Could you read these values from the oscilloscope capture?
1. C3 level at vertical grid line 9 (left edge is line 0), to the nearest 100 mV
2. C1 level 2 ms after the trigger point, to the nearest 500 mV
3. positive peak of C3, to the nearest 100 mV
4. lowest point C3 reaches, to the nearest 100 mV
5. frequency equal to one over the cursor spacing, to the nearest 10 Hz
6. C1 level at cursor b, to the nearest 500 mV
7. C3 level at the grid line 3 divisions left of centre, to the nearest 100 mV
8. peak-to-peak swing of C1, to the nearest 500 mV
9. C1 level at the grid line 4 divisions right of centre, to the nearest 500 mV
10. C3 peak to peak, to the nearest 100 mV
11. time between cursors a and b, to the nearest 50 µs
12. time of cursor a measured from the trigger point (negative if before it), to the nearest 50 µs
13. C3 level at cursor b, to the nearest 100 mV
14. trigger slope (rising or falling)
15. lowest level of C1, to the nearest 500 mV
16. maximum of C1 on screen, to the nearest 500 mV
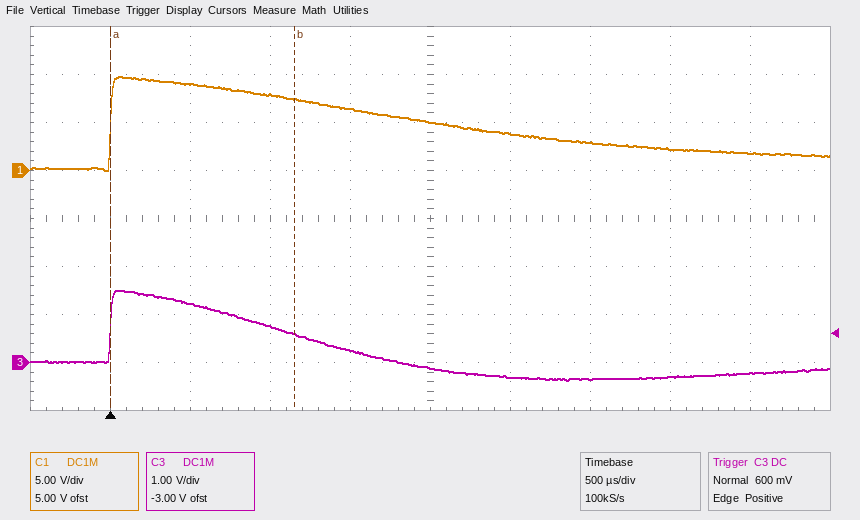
-200 mV
5.0 V
1.5 V
-400 mV
870 Hz
7.5 V
1.2 V
10.0 V
2.0 V
1.9 V
1.15 ms
0 µs
600 mV
rising
0.0 V
10.0 V
